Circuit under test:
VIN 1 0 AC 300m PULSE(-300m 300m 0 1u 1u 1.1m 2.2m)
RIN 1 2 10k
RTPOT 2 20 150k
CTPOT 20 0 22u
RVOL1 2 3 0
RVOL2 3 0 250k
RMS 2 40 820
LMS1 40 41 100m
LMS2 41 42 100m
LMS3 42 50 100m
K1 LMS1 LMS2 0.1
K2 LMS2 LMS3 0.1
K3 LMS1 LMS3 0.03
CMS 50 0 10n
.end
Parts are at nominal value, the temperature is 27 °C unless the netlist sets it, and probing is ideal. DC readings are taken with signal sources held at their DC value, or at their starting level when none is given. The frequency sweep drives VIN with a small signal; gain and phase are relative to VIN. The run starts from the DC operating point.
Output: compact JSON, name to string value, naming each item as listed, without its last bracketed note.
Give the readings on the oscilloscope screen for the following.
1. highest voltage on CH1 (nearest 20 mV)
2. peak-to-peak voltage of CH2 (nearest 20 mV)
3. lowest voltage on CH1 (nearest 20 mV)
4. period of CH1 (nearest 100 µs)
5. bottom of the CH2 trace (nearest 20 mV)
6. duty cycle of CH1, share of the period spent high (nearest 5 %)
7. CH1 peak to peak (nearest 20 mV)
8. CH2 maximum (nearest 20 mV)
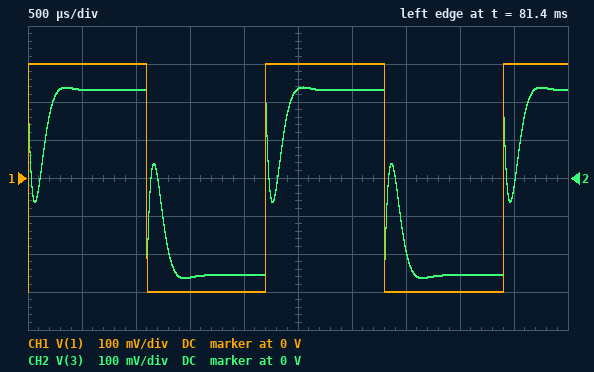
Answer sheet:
{"highest voltage on CH1": "300 mV", "peak-to-peak voltage of CH2": "500 mV", "lowest voltage on CH1": "-300 mV", "period of CH1": "2.2 ms", "bottom of the CH2 trace": "-260 mV", "duty cycle of CH1, share of the period spent high": "50 %", "CH1 peak to peak": "600 mV", "CH2 maximum": "240 mV"}
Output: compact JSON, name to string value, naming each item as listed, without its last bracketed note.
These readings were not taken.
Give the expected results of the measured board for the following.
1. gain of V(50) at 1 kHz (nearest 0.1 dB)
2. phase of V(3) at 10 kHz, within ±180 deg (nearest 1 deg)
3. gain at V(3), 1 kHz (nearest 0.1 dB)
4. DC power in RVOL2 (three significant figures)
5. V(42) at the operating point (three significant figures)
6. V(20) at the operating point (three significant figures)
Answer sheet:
{"gain of V(50) at 1 kHz": "-2.1 dB", "phase of V(3) at 10 kHz, within ±180 deg": "22 deg", "gain at V(3), 1 kHz": "-3.3 dB", "DC power in RVOL2": "237 nW", "V(42) at the operating point": "-243 mV", "V(20) at the operating point": "-243 mV"}
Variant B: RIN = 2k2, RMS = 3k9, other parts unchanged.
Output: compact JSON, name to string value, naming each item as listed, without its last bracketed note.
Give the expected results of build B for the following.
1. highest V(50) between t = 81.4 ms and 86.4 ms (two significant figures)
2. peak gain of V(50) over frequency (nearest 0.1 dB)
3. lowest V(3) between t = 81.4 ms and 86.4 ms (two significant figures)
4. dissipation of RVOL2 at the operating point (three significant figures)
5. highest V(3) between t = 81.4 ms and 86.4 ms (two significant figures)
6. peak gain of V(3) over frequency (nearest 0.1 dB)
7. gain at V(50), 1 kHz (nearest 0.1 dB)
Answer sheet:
{"highest V(50) between t = 81.4 ms and 86.4 ms": "370 mV", "peak gain of V(50) over frequency": "0.7 dB", "lowest V(3) between t = 81.4 ms and 86.4 ms": "-310 mV", "dissipation of RVOL2 at the operating point": "328 nW", "highest V(3) between t = 81.4 ms and 86.4 ms": "300 mV", "peak gain of V(3) over frequency": "-0.4 dB", "gain at V(50), 1 kHz": "0.1 dB"}
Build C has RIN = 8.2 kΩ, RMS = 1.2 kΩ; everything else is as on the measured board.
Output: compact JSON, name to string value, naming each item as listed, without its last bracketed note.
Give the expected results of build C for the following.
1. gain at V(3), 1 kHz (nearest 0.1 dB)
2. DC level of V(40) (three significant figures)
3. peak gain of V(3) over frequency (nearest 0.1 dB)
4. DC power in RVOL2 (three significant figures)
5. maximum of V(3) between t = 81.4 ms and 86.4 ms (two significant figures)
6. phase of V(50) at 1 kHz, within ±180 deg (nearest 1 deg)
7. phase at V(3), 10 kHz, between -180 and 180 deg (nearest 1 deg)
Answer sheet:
{"gain at V(3), 1 kHz": "-2.7 dB", "DC level of V(40)": "-255 mV", "peak gain of V(3) over frequency": "-1.4 dB", "DC power in RVOL2": "261 nW", "maximum of V(3) between t = 81.4 ms and 86.4 ms": "260 mV", "phase of V(50) at 1 kHz, within ±180 deg": "-31 deg", "phase at V(3), 10 kHz, between -180 and 180 deg": "19 deg"}
